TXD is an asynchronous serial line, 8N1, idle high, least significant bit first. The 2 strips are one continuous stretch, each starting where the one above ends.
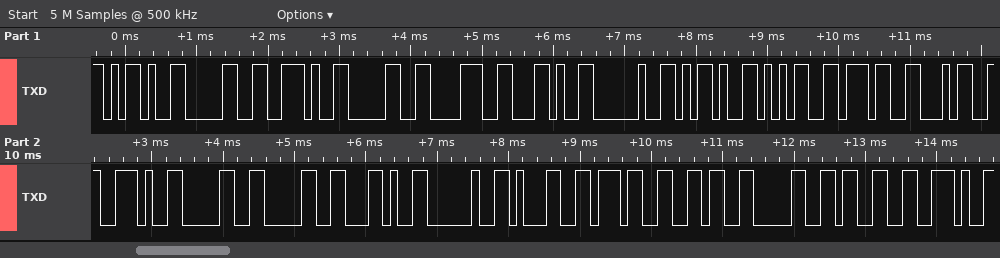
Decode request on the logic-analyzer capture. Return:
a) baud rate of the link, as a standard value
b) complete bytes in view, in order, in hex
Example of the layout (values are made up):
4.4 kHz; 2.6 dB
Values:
9600 baud; 2D 30 2E 30 38 2C 20 2D 35 37 34 2E 30 30 2C 20 31 37 36 30 33 2E
